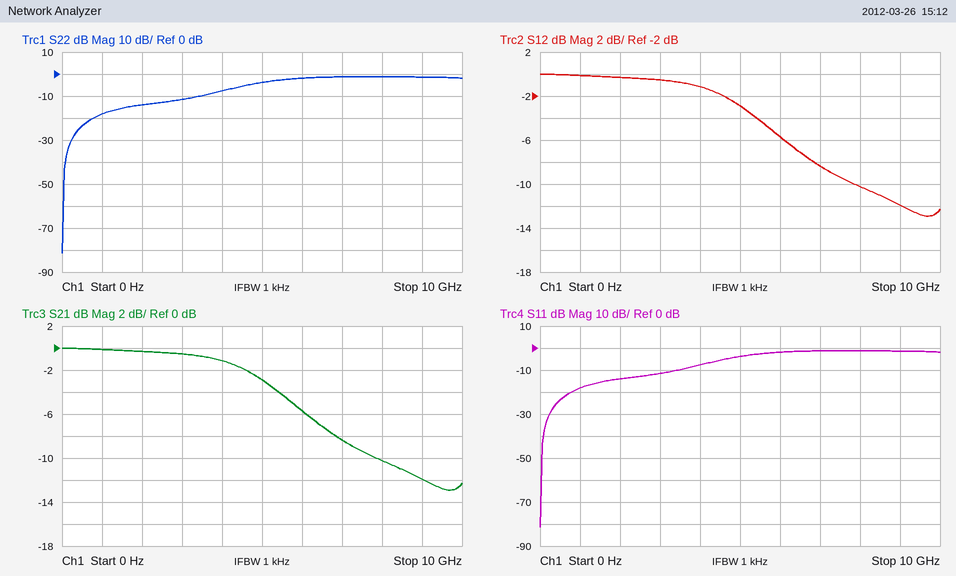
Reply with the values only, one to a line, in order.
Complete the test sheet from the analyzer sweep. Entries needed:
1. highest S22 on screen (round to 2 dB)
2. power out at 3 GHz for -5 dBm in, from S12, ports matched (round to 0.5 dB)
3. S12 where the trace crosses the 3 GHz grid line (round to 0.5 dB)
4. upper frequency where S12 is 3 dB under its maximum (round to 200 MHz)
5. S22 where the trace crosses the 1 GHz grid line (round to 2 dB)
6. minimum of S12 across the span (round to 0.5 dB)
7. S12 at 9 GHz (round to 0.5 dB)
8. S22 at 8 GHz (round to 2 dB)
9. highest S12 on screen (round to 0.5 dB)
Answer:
-2 dB
-5.5 dBm
-0.5 dB
5.0 GHz
-18 dB
-13.0 dB
-12.0 dB
-2 dB
0.0 dB
